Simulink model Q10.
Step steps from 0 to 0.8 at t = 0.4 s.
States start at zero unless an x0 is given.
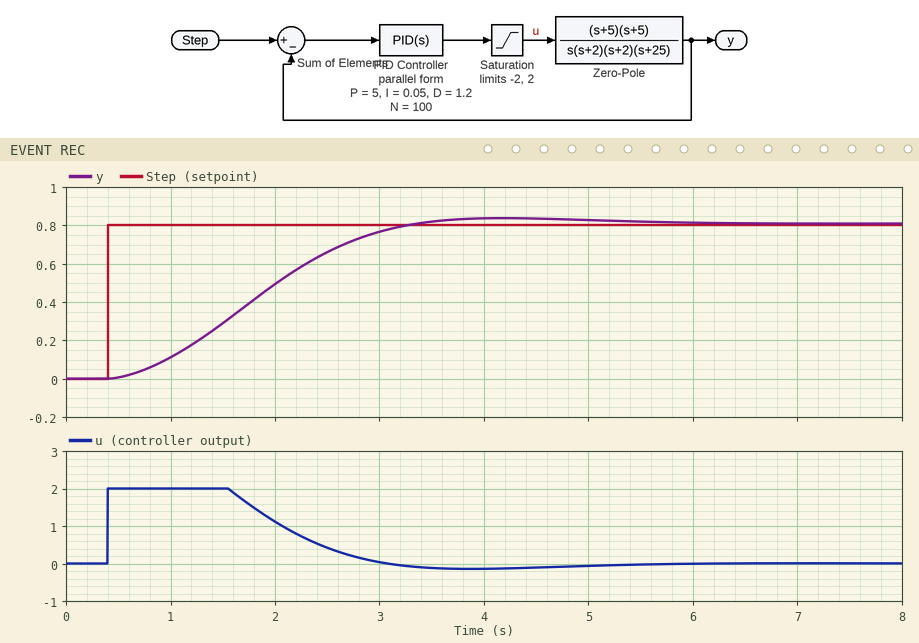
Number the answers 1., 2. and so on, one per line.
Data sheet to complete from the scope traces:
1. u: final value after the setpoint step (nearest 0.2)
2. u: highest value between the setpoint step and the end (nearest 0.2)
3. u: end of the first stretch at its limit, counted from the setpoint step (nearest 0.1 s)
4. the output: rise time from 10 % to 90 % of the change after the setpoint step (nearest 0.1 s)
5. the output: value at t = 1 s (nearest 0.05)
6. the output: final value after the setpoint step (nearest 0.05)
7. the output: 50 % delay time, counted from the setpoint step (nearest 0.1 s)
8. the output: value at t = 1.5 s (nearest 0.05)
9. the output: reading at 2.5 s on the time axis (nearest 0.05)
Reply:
1. 0.0
2. 2.0
3. 1.2 s
4. 1.9 s
5. 0.10
6. 0.80
7. 1.4 s
8. 0.30
9. 0.65
